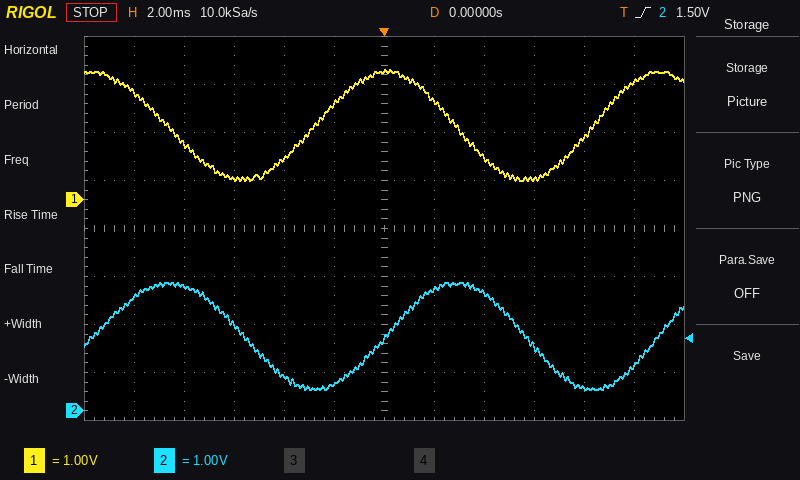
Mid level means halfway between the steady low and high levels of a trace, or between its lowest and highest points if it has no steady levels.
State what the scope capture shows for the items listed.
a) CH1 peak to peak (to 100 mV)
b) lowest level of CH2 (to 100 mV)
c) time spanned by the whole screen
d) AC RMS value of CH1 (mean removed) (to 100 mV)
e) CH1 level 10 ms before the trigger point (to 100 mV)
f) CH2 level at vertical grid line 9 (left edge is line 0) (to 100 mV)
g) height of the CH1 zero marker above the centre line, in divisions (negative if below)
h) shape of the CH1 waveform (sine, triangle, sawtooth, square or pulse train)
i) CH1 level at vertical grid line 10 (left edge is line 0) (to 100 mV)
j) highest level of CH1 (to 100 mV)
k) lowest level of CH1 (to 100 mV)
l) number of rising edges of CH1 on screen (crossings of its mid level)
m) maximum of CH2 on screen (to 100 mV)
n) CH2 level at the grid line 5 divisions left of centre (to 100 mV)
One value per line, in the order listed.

2.3 V
400 mV
24 ms
800 mV
2.2 V
1.3 V
+0.6 div
sine
1.3 V
2.7 V
400 mV
2
2.7 V
2.4 V
